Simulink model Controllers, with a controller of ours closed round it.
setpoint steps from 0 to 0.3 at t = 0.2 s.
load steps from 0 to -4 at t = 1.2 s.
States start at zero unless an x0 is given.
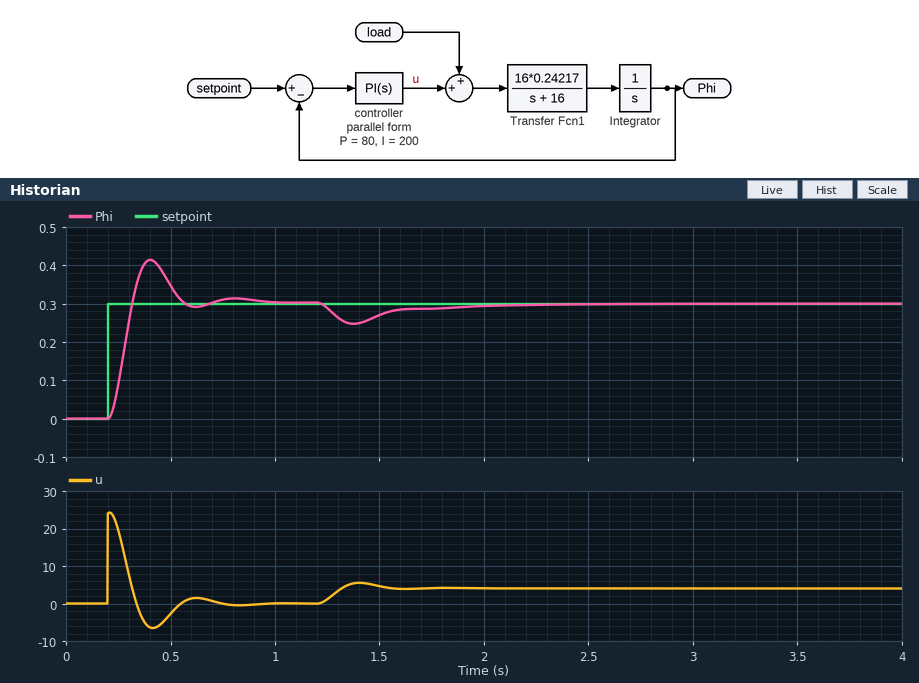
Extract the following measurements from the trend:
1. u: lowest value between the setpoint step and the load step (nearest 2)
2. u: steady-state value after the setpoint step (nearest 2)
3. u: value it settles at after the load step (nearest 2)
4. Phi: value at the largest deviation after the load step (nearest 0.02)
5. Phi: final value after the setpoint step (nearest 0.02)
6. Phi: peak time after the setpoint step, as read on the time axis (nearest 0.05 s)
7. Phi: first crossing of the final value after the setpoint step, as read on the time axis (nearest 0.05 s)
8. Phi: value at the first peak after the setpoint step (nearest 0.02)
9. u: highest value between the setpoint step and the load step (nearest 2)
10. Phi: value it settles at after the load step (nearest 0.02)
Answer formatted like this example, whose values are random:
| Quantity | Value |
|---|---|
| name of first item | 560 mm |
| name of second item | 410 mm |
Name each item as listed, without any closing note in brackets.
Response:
| Quantity | Value |
|---|---|
| u: lowest value between the setpoint step and the load step | -6 |
| u: steady-state value after the setpoint step | 0 |
| u: value it settles at after the load step | 4 |
| Phi: value at the largest deviation after the load step | 0.24 |
| Phi: final value after the setpoint step | 0.30 |
| Phi: peak time after the setpoint step, as read on the time axis | 0.40 s |
| Phi: first crossing of the final value after the setpoint step, as read on the time axis | 0.30 s |
| Phi: value at the first peak after the setpoint step | 0.42 |
| u: highest value between the setpoint step and the load step | 24 |
| Phi: value it settles at after the load step | 0.30 |
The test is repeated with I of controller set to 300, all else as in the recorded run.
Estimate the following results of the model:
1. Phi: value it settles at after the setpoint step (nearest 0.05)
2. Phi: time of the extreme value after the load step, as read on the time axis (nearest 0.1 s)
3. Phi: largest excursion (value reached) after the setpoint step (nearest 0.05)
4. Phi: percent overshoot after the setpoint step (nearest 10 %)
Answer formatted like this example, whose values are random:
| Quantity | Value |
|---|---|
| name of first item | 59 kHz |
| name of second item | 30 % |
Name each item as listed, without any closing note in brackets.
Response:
| Quantity | Value |
|---|---|
| Phi: value it settles at after the setpoint step | 0.30 |
| Phi: time of the extreme value after the load step, as read on the time axis | 1.4 s |
| Phi: largest excursion (value reached) after the setpoint step | 0.45 |
| Phi: percent overshoot after the setpoint step | 50 % |
